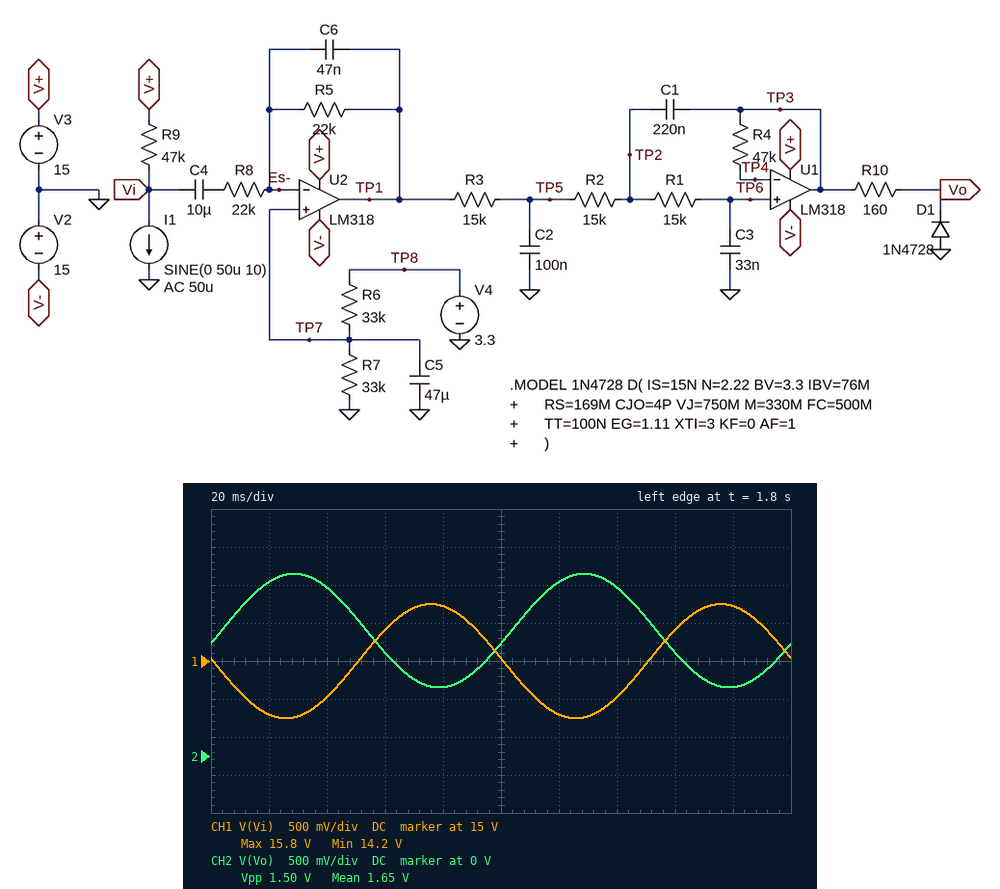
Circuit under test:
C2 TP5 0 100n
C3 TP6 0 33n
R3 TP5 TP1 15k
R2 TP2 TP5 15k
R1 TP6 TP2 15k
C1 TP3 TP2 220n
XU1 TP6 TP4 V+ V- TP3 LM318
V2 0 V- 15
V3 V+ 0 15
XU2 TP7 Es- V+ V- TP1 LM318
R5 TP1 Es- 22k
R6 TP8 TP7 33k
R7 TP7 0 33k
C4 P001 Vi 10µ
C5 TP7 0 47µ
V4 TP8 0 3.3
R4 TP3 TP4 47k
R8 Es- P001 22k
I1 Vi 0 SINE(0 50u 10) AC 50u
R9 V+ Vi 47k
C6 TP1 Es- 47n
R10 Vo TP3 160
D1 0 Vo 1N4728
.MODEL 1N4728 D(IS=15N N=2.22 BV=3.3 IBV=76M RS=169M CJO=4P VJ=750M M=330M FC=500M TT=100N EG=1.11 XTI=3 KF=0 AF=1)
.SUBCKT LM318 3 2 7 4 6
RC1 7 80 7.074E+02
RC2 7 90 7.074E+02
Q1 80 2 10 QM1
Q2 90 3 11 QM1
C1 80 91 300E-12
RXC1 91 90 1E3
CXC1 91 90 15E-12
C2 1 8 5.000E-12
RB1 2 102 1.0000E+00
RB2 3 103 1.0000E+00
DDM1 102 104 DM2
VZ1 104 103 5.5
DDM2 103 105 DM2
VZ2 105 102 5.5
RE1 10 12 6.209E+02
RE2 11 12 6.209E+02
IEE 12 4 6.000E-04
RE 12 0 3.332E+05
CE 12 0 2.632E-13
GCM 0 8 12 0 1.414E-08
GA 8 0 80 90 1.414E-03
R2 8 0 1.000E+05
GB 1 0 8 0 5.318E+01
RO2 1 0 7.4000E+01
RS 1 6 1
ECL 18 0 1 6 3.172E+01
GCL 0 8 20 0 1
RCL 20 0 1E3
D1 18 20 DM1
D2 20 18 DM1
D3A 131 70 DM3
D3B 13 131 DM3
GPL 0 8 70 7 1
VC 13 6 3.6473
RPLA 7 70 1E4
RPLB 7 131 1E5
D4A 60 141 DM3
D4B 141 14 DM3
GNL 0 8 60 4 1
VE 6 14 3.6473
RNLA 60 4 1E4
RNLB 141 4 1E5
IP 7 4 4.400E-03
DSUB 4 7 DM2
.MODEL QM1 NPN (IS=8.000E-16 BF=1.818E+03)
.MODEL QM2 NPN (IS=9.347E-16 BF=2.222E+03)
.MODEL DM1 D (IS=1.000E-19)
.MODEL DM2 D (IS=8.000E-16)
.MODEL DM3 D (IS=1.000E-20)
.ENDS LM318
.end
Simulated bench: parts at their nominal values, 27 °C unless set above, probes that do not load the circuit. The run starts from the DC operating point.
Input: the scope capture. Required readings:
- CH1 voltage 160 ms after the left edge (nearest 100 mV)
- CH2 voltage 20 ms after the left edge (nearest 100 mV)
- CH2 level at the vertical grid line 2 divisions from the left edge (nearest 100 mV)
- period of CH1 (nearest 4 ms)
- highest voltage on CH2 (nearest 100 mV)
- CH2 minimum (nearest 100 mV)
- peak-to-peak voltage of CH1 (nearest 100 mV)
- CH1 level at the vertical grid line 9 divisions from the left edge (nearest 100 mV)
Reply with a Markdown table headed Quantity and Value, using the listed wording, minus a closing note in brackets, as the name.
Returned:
| Quantity | Value |
|---|---|
| CH1 voltage 160 ms after the left edge | 15.4 V |
| CH2 voltage 20 ms after the left edge | 2.3 V |
| CH2 level at the vertical grid line 2 divisions from the left edge | 2.2 V |
| period of CH1 | 100 ms |
| highest voltage on CH2 | 2.4 V |
| CH2 minimum | 900 mV |
| peak-to-peak voltage of CH1 | 1.5 V |
| CH1 level at the vertical grid line 9 divisions from the left edge | 15.7 V |
